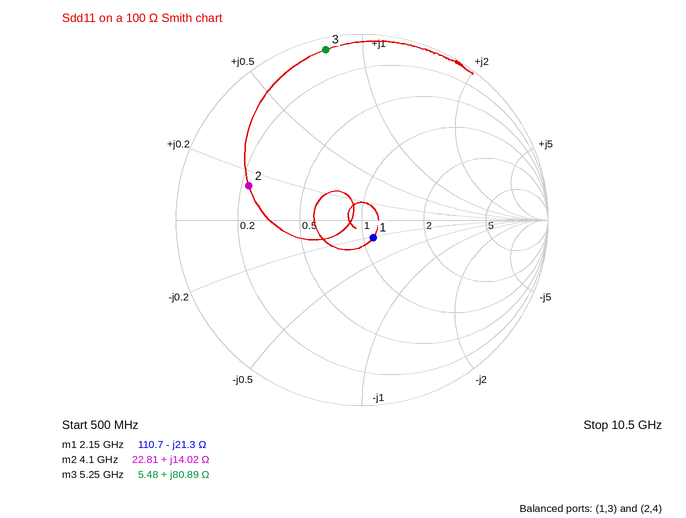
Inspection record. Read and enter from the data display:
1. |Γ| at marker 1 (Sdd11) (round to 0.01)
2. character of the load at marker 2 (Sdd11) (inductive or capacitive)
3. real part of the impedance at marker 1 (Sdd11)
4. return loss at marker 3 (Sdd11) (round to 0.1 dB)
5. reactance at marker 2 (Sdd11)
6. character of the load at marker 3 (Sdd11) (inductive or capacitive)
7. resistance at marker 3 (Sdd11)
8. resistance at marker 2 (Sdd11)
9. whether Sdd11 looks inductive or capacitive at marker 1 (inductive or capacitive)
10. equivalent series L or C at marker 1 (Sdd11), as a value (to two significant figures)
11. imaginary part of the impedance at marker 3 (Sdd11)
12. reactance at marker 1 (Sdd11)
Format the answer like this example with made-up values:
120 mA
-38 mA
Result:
0.11
inductive
110.7 Ω
0.6 dB
+14.02 Ω
inductive
5.48 Ω
22.81 Ω
capacitive
3.5 pF
+80.89 Ω
-21.3 Ω
